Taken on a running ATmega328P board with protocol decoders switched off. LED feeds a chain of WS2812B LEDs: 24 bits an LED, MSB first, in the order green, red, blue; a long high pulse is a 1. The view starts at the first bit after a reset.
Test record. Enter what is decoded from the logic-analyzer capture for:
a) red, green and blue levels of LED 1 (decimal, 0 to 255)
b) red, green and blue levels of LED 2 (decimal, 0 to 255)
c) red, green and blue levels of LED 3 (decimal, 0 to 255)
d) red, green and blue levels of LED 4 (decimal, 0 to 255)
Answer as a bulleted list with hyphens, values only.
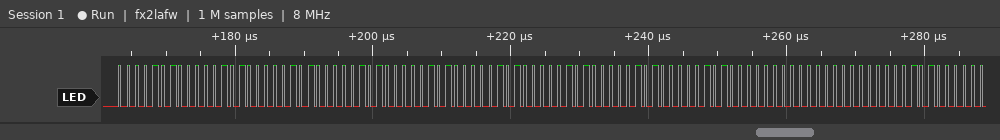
- 10, 10, 10
- 10, 10, 10
- 10, 10, 10
- 0, 0, 10
